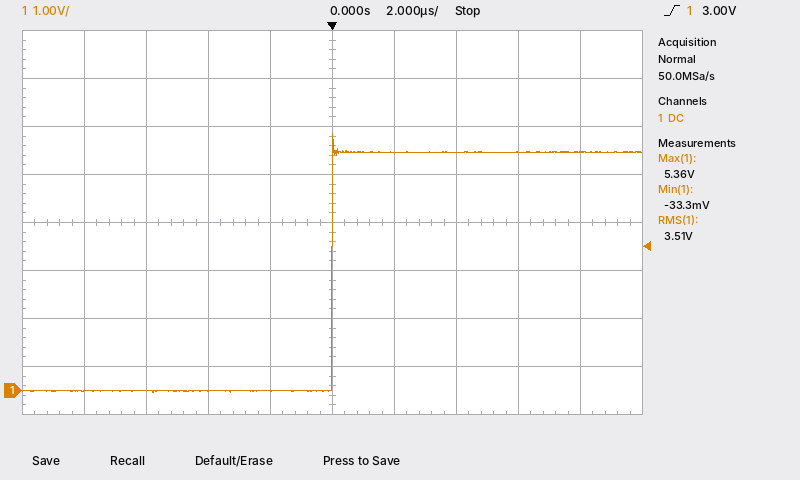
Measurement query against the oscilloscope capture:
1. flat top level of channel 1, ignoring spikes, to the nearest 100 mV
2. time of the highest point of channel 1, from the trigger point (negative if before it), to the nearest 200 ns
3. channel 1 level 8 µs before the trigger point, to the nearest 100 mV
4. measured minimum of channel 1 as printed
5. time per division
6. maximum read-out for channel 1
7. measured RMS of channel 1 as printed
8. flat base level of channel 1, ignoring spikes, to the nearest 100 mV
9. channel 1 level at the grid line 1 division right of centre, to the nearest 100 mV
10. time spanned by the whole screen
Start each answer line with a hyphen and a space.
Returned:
- 5.0 V
- 0.0 µs
- 0.0 V
- -33.3 mV
- 2 µs
- 5.36 V
- 3.51 V
- 0.0 V
- 5.0 V
- 20 µs
